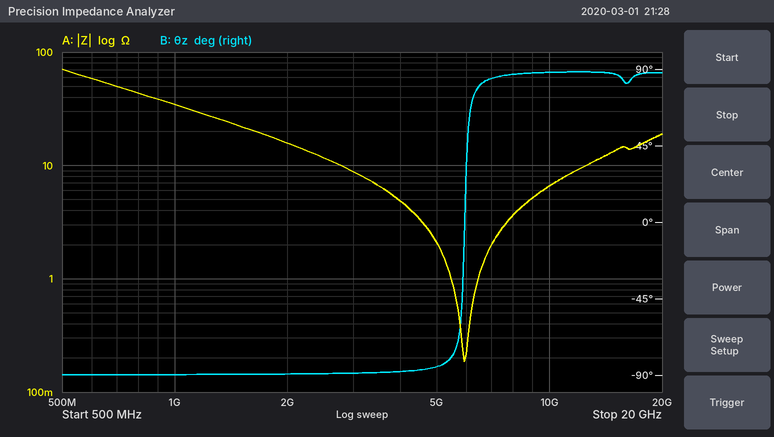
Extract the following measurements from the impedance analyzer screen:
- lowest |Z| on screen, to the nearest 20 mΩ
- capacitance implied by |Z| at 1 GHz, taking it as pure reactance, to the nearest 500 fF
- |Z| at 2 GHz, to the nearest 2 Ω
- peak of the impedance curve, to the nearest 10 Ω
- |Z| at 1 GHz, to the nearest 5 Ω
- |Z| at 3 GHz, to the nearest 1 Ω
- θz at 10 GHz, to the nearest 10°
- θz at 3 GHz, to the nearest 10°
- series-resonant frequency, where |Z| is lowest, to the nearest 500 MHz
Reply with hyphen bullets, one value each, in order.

- 180 mΩ
- 4.5 pF
- 16 Ω
- 70 Ω
- 35 Ω
- 9 Ω
- 90°
- -90°
- 6.0 GHz
